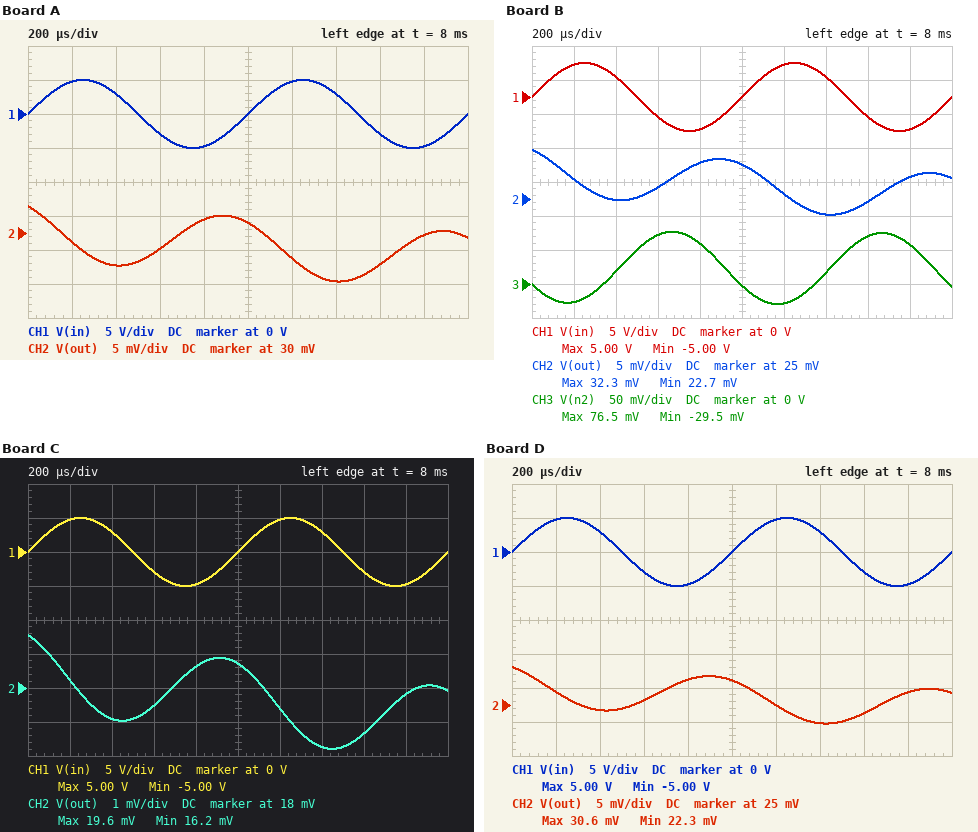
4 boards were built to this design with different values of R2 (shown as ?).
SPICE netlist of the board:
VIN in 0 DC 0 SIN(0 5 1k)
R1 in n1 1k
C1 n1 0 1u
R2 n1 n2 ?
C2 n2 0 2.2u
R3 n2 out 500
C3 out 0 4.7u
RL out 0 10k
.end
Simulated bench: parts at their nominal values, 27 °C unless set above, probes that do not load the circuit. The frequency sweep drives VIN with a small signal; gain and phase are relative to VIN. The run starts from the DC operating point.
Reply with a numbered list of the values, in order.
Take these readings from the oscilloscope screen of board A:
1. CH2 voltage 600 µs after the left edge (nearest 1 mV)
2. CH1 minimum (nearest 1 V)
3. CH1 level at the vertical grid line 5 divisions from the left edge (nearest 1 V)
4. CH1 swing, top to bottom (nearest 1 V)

1. 28 mV
2. -5 V
3. 0 V
4. 10 V
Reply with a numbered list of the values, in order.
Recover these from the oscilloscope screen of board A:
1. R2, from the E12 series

1. 820 Ω
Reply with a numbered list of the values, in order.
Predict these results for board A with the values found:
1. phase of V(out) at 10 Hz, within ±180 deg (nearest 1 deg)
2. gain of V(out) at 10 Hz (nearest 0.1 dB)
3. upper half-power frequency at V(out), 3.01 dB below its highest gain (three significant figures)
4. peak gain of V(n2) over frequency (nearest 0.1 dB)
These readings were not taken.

1. -41 deg
2. -3.8 dB
3. 13.2 Hz
4. -1.4 dB
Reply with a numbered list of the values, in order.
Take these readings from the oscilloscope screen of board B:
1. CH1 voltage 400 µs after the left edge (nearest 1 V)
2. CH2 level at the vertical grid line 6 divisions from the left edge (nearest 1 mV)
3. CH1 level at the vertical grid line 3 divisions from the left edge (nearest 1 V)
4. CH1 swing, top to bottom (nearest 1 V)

1. 3 V
2. 26 mV
3. -3 V
4. 10 V
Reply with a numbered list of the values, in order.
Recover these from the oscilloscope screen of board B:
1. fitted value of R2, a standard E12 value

1. 1 kΩ
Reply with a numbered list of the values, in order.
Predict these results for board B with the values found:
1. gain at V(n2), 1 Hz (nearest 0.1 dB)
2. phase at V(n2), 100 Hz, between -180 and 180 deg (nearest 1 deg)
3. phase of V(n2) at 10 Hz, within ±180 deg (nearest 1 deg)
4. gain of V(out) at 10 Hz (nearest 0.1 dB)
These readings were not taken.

1. -1.5 dB
2. -69 deg
3. -35 deg
4. -4.1 dB
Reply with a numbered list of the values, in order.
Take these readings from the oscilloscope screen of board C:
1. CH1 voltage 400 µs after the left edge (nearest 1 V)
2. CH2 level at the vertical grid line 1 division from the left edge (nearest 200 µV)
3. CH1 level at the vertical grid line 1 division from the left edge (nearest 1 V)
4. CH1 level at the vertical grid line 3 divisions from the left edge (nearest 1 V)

1. 3 V
2. 18.2 mV
3. 5 V
4. -3 V
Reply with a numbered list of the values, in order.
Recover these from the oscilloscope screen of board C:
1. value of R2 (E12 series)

1. 3.3 kΩ
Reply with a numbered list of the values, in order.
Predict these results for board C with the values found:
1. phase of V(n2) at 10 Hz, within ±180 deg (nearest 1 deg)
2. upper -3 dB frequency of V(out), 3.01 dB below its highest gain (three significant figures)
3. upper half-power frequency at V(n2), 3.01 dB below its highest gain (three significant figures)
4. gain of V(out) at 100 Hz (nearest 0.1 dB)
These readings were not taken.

1. -51 deg
2. 7.42 Hz
3. 7.50 Hz
4. -27.7 dB
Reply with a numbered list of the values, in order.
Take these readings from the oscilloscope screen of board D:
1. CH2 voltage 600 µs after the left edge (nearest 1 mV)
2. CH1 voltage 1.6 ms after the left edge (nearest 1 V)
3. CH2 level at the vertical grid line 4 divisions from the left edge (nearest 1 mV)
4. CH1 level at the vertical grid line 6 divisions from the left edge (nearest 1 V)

1. 26 mV
2. -3 V
3. 29 mV
4. 5 V
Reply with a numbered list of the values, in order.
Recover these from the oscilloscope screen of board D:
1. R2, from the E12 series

1. 1.2 kΩ
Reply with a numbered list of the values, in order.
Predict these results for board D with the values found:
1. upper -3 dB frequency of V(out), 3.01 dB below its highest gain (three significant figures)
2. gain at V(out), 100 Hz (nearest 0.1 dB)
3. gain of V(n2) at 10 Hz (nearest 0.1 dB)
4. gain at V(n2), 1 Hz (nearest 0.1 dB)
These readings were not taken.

1. 11.6 Hz
2. -22.1 dB
3. -4.0 dB
4. -1.7 dB
